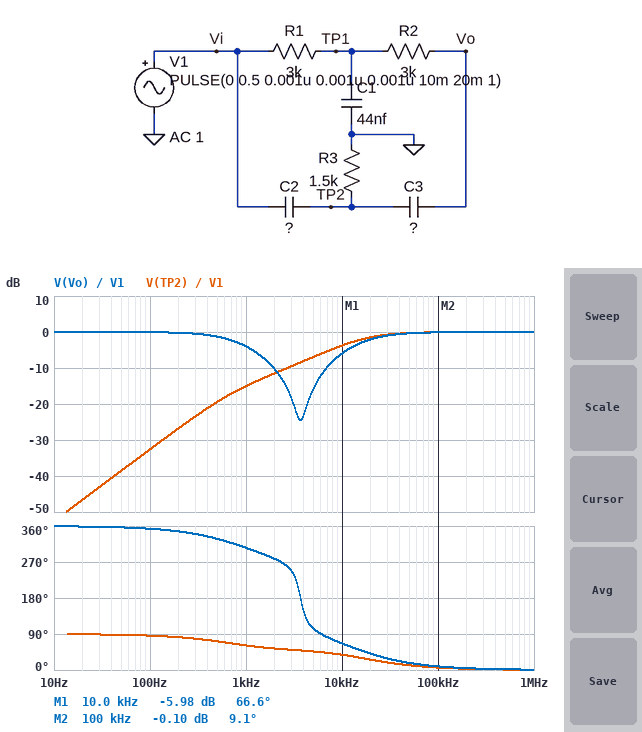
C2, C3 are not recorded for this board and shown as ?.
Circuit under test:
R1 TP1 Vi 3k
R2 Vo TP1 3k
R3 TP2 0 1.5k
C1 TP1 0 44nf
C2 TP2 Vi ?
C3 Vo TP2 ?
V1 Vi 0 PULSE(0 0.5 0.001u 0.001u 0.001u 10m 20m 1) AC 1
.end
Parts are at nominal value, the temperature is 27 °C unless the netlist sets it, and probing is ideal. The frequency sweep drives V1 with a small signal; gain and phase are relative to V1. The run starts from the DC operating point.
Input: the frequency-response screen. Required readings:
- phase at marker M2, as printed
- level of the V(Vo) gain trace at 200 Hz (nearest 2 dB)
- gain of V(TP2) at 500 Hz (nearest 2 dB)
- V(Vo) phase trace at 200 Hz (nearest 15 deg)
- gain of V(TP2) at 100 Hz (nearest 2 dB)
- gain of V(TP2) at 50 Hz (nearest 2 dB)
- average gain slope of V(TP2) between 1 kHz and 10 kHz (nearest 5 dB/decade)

9.1 deg
0 dB
-20 dB
345 deg
-32 dB
-38 dB
10 dB/decade
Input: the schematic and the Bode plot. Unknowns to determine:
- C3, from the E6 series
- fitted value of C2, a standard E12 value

10 nF
15 nF
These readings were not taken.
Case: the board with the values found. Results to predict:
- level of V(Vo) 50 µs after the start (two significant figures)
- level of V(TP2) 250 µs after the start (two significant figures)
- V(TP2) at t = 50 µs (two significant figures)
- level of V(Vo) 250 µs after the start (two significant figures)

57 mV
16 mV
78 mV
360 mV
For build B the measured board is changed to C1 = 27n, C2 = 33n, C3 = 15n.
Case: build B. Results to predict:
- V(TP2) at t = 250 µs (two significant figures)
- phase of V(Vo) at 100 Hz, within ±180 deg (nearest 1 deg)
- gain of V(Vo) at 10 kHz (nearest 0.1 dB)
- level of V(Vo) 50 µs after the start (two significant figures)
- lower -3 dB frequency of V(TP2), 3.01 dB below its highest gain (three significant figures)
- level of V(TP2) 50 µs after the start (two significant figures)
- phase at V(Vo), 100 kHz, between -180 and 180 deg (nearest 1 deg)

34 mV
-6 deg
-3.0 dB
120 mV
5.23 kHz
180 mV
5 deg
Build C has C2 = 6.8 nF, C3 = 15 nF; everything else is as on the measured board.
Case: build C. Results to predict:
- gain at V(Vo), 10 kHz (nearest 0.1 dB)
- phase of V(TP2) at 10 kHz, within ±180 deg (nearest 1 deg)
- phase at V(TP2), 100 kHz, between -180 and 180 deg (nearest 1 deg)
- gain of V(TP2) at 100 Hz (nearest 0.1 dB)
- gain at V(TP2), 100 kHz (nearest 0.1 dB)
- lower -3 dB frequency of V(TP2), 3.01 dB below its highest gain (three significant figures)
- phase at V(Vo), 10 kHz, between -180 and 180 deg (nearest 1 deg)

-10.3 dB
57 deg
13 deg
-33.8 dB
-0.3 dB
25.4 kHz
80 deg
